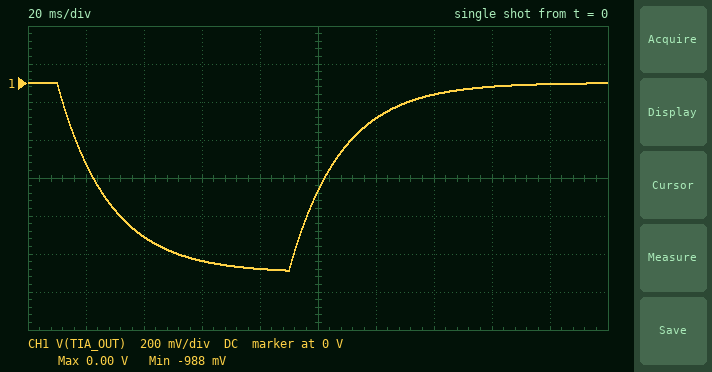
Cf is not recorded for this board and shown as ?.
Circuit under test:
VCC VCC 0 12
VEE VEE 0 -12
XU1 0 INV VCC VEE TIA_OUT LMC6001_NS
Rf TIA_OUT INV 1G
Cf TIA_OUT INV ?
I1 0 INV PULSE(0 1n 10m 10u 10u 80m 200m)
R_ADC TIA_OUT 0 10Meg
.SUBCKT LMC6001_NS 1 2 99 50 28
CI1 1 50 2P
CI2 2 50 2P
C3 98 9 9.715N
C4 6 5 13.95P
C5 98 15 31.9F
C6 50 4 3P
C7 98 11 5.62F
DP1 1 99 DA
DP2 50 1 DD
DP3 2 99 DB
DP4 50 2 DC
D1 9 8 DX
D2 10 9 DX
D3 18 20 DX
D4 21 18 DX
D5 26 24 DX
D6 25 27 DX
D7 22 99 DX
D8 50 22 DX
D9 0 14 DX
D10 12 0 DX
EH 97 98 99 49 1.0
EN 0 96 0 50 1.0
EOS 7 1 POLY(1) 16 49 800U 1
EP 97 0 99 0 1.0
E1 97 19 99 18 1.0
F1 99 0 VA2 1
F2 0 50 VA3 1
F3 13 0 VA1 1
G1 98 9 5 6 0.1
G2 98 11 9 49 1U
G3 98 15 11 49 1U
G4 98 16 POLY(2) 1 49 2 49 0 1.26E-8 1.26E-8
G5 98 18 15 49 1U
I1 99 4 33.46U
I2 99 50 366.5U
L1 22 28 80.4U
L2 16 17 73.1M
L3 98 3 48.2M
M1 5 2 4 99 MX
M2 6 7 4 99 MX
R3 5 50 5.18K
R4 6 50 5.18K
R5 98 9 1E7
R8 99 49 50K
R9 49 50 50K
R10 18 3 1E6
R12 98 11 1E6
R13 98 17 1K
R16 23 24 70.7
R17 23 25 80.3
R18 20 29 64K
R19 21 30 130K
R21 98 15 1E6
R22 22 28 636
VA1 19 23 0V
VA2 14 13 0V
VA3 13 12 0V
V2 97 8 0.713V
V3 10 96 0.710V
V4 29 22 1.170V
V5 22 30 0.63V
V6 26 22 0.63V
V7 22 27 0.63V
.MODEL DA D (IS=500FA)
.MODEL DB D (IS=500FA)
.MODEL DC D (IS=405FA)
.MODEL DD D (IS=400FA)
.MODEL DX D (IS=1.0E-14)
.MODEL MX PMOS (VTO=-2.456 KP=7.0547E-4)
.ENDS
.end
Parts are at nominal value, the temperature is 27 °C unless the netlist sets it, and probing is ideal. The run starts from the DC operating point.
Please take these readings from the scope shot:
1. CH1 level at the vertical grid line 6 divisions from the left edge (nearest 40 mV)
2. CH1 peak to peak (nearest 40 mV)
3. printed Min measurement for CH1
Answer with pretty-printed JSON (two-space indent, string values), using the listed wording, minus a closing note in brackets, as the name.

{
  "CH1 level at the vertical grid line 6 divisions from the left edge": "-200 mV",
  "CH1 peak to peak": "1.00 V",
  "printed Min measurement for CH1": "-988 mV"
}
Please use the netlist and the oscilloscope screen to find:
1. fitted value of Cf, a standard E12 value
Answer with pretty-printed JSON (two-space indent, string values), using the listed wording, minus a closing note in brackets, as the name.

{
  "fitted value of Cf, a standard E12 value": "18 pF"
}
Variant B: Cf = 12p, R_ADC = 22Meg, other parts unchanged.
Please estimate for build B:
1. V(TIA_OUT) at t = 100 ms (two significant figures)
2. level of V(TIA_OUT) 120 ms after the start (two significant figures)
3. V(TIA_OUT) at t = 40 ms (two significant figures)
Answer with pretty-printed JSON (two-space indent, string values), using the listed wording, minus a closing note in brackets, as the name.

{
  "V(TIA_OUT) at t = 100 ms": "-430 mV",
  "level of V(TIA_OUT) 120 ms after the start": "-81 mV",
  "V(TIA_OUT) at t = 40 ms": "-920 mV"
}
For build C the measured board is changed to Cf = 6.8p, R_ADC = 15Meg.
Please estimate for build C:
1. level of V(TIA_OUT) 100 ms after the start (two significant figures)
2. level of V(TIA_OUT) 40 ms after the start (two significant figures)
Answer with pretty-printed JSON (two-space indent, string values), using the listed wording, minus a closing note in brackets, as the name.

{
  "level of V(TIA_OUT) 100 ms after the start": "-230 mV",
  "level of V(TIA_OUT) 40 ms after the start": "-990 mV"
}
